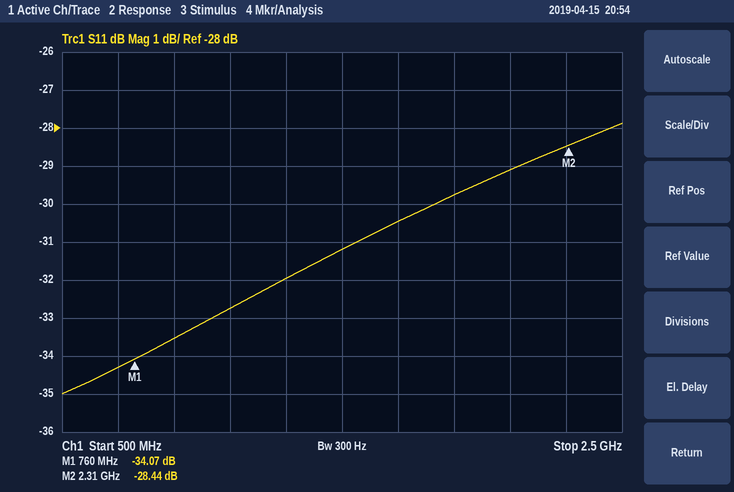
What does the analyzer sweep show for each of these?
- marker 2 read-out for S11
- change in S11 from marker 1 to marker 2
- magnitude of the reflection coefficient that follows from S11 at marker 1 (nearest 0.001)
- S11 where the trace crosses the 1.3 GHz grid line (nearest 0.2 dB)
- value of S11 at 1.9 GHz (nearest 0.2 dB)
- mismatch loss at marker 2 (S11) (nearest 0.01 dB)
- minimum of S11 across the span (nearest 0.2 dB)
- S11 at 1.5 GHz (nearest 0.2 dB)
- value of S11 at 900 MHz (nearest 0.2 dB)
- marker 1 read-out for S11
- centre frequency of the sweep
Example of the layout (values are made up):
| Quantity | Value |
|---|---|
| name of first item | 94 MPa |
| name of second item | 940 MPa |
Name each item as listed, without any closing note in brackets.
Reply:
| Quantity | Value |
|---|---|
| marker 2 read-out for S11 | -28.44 dB |
| change in S11 from marker 1 to marker 2 | 5.63 dB |
| magnitude of the reflection coefficient that follows from S11 at marker 1 | 0.020 |
| S11 where the trace crosses the 1.3 GHz grid line | -32.0 dB |
| value of S11 at 1.9 GHz | -29.8 dB |
| mismatch loss at marker 2 (S11) | 0.01 dB |
| minimum of S11 across the span | -35.0 dB |
| S11 at 1.5 GHz | -31.2 dB |
| value of S11 at 900 MHz | -33.6 dB |
| marker 1 read-out for S11 | -34.07 dB |
| centre frequency of the sweep | 1.5 GHz |
